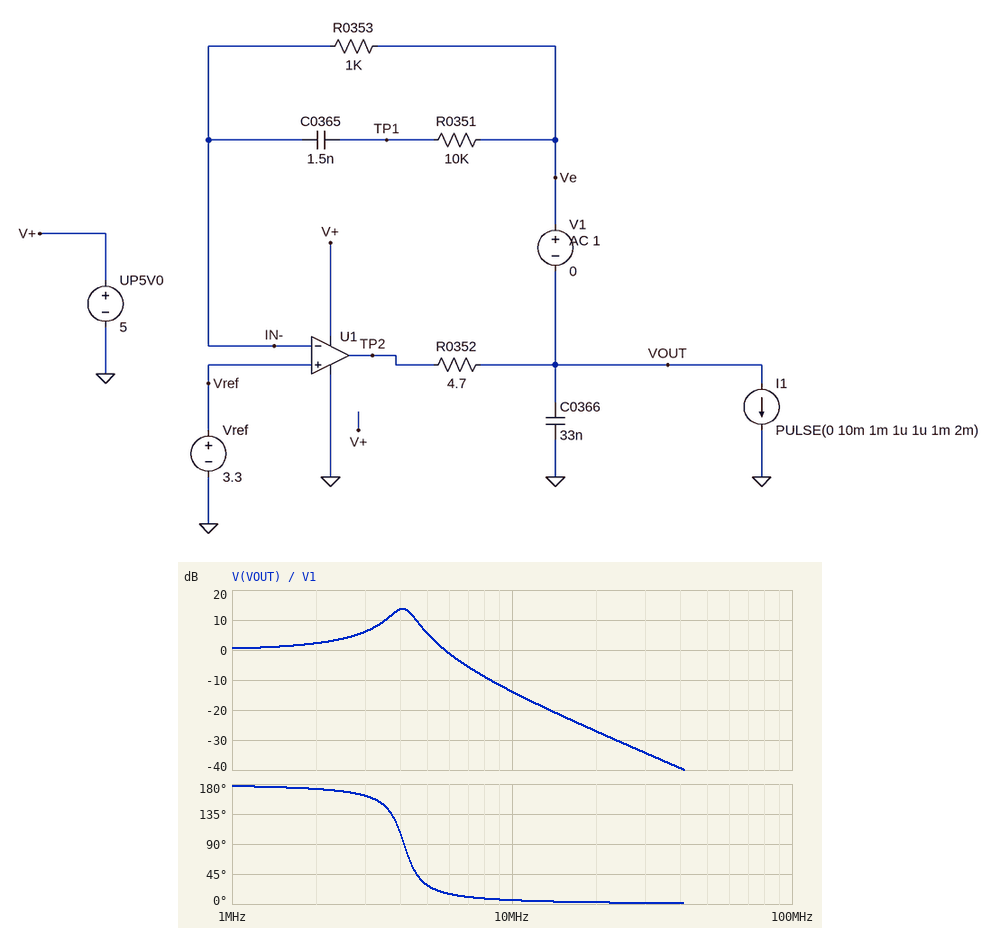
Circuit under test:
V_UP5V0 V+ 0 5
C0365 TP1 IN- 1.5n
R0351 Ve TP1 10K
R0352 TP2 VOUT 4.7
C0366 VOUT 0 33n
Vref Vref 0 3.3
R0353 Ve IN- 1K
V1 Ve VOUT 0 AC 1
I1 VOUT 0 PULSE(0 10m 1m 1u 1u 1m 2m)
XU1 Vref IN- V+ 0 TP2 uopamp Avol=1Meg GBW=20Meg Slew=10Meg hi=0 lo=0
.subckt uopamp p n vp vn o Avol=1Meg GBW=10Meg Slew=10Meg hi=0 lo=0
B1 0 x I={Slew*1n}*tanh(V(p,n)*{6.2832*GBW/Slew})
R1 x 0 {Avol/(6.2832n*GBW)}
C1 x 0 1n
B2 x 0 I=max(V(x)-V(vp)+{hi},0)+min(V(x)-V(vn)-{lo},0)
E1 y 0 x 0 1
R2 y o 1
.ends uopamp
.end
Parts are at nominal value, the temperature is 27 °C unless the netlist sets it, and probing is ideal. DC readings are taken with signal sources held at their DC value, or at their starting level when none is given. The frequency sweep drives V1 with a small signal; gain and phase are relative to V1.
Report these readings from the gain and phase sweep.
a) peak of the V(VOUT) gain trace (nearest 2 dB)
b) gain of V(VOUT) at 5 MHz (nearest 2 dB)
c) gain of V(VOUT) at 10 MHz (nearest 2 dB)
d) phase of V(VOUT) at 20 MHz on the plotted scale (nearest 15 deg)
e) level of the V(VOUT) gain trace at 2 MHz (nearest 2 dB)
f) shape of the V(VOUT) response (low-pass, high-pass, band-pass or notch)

14 dB
6 dB
-14 dB
0 deg
2 dB
low-pass
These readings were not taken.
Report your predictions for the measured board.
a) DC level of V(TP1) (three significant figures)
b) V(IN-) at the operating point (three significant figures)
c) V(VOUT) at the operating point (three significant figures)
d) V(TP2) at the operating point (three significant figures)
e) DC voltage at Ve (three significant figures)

3.30 V
3.30 V
3.30 V
3.30 V
3.30 V
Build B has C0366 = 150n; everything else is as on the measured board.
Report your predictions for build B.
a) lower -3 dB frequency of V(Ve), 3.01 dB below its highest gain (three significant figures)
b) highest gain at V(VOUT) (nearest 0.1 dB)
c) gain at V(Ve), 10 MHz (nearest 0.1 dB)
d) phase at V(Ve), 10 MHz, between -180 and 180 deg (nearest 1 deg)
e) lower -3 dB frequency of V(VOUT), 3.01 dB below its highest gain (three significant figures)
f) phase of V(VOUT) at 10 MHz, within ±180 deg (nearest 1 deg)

1.85 MHz
20.3 dB
0.3 dB
0 deg
1.83 MHz
1 deg
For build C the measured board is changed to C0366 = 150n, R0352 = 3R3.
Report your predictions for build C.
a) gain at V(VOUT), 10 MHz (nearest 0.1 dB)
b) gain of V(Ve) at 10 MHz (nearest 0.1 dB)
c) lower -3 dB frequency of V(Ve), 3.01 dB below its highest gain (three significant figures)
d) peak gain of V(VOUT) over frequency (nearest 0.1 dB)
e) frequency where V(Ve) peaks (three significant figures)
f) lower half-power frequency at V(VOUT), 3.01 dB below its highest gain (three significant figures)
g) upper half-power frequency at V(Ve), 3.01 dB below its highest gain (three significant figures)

-25.7 dB
0.4 dB
2.11 MHz
19.1 dB
2.23 MHz
2.09 MHz
2.36 MHz
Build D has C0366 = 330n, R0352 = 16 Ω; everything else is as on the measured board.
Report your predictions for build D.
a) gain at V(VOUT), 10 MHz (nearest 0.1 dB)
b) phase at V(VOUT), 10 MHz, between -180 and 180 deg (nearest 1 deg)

-44.9 dB
0 deg
